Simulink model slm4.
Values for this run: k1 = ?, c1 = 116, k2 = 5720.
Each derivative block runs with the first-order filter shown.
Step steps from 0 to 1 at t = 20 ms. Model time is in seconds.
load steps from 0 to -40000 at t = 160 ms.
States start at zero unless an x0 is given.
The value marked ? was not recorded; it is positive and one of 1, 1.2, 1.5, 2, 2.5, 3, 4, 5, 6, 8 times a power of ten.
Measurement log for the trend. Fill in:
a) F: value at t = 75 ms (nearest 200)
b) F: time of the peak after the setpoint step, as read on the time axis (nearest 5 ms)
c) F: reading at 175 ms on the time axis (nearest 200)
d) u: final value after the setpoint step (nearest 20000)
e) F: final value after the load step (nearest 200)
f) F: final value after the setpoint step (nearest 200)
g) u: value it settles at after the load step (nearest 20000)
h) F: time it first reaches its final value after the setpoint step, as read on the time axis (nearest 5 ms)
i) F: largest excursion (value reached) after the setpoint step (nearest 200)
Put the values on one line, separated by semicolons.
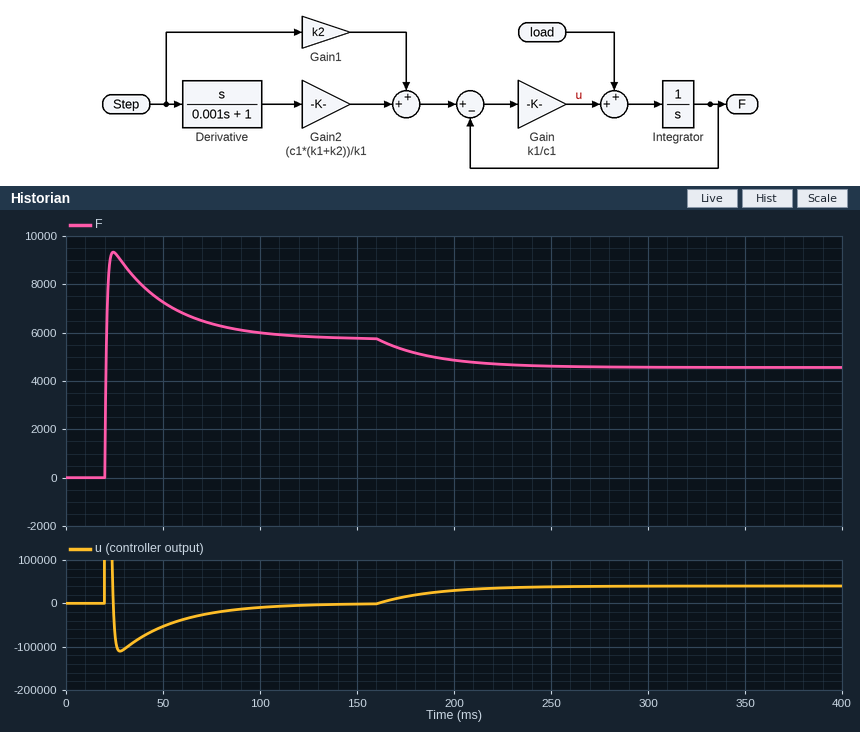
6400; 25 ms; 5200; 0; 4600; 5800; 40000; 20 ms; 9400
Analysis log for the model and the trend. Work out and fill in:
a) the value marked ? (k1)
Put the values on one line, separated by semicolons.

4000
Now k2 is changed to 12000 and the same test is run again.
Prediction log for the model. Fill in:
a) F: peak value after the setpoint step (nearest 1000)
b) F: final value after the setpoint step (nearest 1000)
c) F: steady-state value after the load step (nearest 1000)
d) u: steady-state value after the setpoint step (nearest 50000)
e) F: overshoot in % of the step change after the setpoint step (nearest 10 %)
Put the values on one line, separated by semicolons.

16000; 12000; 11000; 0; 30 %
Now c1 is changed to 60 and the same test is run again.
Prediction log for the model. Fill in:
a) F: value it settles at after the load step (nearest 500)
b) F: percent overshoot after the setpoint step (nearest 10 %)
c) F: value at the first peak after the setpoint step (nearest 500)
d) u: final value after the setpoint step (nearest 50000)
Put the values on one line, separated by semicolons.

5000; 60 %; 9000; 0
